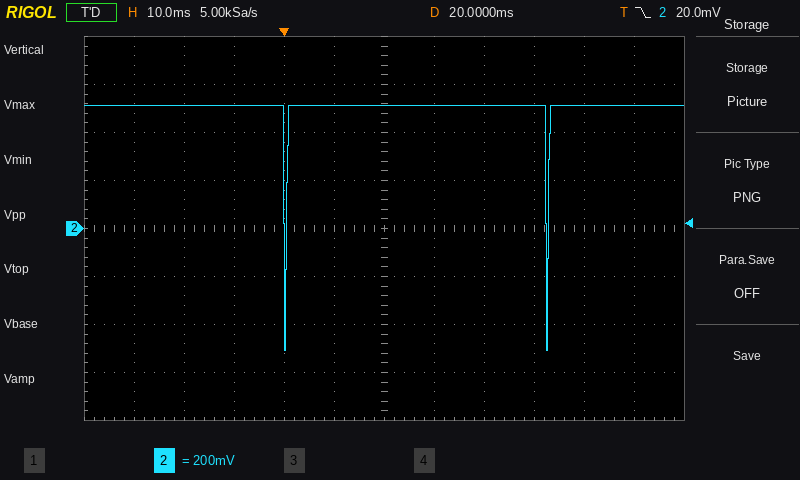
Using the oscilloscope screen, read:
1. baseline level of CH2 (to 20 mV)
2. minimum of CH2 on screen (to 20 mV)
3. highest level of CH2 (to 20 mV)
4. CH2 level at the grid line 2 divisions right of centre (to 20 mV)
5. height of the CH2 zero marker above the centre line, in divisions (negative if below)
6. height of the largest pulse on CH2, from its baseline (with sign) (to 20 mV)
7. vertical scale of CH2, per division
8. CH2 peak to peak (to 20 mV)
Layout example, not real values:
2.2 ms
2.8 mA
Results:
520 mV
-500 mV
520 mV
520 mV
0.0 div
-1.02 V
200 mV
1.02 V
